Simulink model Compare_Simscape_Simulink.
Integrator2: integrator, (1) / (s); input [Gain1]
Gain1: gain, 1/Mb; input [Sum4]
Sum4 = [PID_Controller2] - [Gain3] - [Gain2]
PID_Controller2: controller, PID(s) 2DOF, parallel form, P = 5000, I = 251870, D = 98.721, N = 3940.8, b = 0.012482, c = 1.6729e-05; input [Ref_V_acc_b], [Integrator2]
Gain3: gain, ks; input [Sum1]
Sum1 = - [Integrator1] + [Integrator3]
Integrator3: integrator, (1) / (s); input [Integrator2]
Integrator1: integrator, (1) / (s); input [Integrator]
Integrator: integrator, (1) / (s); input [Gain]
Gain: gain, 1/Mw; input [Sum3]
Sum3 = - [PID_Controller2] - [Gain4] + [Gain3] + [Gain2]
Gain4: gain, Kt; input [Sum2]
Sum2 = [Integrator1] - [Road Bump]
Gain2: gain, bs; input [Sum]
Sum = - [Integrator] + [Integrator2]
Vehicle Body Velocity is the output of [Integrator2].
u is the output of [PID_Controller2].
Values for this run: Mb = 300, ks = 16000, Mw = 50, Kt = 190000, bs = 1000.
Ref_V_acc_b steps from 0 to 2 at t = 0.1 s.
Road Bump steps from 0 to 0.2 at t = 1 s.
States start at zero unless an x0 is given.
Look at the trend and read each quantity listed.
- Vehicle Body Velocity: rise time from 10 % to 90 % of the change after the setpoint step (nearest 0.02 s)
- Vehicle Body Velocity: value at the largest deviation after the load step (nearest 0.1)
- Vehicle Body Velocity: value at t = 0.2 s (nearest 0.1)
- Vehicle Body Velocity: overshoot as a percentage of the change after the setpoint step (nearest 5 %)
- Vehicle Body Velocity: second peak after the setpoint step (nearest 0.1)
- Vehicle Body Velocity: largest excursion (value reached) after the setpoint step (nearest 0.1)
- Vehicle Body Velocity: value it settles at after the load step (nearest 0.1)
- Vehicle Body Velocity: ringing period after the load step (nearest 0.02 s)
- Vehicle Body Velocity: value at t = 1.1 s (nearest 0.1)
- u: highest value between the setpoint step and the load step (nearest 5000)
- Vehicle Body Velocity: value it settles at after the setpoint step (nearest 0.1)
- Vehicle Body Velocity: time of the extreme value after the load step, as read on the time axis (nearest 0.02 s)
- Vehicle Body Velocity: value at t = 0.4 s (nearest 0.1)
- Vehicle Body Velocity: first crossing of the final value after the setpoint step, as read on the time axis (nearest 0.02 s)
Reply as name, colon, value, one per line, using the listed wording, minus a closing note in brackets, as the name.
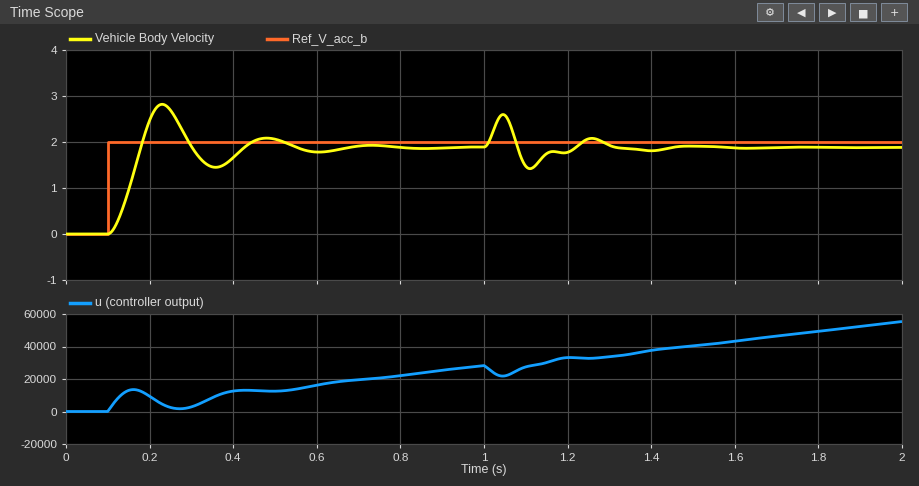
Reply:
Vehicle Body Velocity: rise time from 10 % to 90 % of the change after the setpoint step: 0.06 s
Vehicle Body Velocity: value at the largest deviation after the load step: 2.6
Vehicle Body Velocity: value at t = 0.2 s: 2.5
Vehicle Body Velocity: overshoot as a percentage of the change after the setpoint step: 50 %
Vehicle Body Velocity: second peak after the setpoint step: 2.1
Vehicle Body Velocity: largest excursion (value reached) after the setpoint step: 2.8
Vehicle Body Velocity: value it settles at after the load step: 1.9
Vehicle Body Velocity: ringing period after the load step: 0.22 s
Vehicle Body Velocity: value at t = 1.1 s: 1.5
u: highest value between the setpoint step and the load step: 30000
Vehicle Body Velocity: value it settles at after the setpoint step: 1.9
Vehicle Body Velocity: time of the extreme value after the load step, as read on the time axis: 1.04 s
Vehicle Body Velocity: value at t = 0.4 s: 1.7
Vehicle Body Velocity: first crossing of the final value after the setpoint step, as read on the time axis: 0.18 s
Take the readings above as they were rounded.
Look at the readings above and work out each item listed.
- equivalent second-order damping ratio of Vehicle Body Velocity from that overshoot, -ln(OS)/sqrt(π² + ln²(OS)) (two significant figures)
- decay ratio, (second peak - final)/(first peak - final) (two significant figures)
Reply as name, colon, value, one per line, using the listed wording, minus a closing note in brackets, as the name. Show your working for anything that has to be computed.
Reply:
equivalent second-order damping ratio of Vehicle Body Velocity from that overshoot, -ln(OS)/sqrt(π² + ln²(OS)): ln(0.5) = -0.693; 0.693 / sqrt(9.870 + 0.480) = 0.22
decay ratio, (second peak - final)/(first peak - final): (2.1 - 1.9) / (2.8 - 1.9) = 0.22
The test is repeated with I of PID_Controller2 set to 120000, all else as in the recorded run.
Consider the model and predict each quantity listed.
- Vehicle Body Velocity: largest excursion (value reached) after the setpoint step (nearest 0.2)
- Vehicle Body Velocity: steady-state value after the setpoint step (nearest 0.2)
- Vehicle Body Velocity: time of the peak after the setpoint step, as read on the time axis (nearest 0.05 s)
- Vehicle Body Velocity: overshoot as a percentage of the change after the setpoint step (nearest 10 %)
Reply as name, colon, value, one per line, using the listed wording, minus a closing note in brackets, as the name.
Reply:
Vehicle Body Velocity: largest excursion (value reached) after the setpoint step: 2.2
Vehicle Body Velocity: steady-state value after the setpoint step: 1.8
Vehicle Body Velocity: time of the peak after the setpoint step, as read on the time axis: 0.30 s
Vehicle Body Velocity: overshoot as a percentage of the change after the setpoint step: 30 %
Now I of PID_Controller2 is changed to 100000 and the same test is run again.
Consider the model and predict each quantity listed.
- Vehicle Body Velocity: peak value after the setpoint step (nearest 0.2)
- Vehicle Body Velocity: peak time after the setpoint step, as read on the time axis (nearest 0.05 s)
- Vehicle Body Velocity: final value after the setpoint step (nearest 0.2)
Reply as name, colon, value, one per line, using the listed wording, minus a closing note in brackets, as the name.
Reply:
Vehicle Body Velocity: peak value after the setpoint step: 2.2
Vehicle Body Velocity: peak time after the setpoint step, as read on the time axis: 0.30 s
Vehicle Body Velocity: final value after the setpoint step: 1.8
